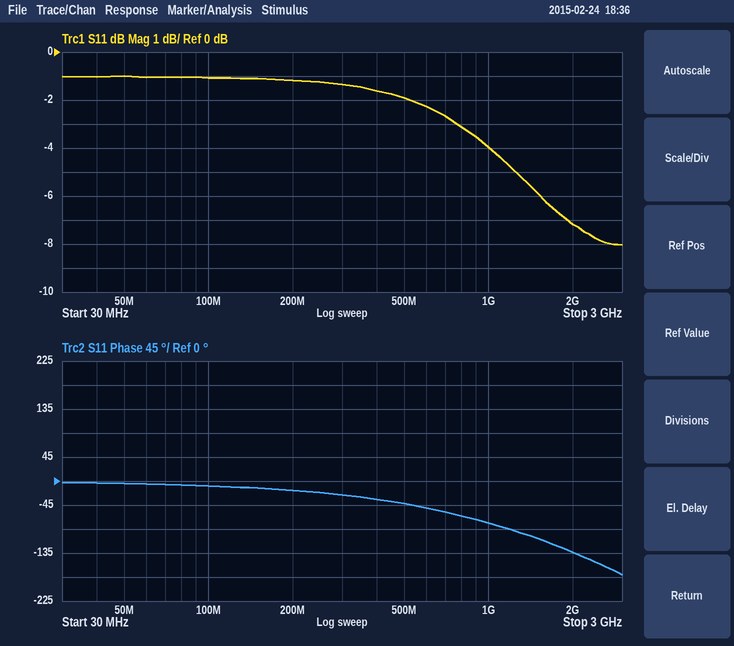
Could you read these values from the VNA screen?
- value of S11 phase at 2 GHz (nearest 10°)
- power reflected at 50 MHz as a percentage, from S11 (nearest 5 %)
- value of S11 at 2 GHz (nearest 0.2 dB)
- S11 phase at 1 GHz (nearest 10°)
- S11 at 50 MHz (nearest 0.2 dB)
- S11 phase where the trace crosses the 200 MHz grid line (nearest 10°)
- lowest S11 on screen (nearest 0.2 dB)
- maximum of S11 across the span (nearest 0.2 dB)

-130°
80 %
-7.2 dB
-80°
-1.0 dB
-20°
-8.0 dB
-1.0 dB
